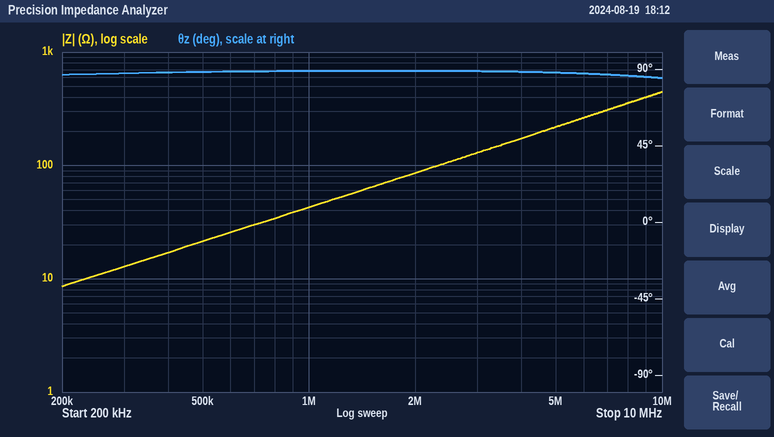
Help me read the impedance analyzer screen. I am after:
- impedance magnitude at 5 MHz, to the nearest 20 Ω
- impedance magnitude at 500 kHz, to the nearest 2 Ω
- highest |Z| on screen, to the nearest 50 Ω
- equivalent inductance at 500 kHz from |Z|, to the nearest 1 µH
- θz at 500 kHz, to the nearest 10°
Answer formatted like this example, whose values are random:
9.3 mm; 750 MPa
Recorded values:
220 Ω; 22 Ω; 450 Ω; 7 µH; 90°
